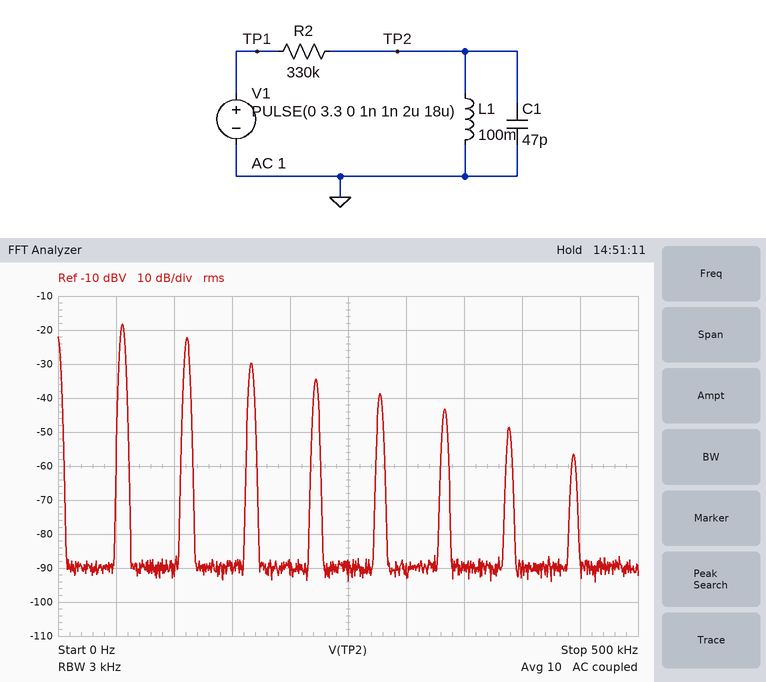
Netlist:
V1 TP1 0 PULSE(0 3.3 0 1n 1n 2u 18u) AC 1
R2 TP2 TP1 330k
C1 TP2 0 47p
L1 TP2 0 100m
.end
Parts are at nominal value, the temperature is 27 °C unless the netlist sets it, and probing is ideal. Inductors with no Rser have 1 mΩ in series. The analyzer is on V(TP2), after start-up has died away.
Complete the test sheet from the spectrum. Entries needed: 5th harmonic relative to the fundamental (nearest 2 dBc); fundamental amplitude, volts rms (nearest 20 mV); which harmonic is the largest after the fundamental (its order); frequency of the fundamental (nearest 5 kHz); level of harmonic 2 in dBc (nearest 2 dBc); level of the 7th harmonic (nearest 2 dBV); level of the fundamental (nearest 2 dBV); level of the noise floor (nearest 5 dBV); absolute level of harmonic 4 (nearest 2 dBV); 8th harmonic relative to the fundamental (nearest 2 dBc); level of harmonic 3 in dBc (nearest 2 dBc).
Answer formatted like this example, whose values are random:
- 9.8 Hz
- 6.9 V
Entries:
- -20 dBc
- 120 mV
- 2
- 55 kHz
- -4 dBc
- -48 dBV
- -18 dBV
- -90 dBV
- -34 dBV
- -38 dBc
- -12 dBc
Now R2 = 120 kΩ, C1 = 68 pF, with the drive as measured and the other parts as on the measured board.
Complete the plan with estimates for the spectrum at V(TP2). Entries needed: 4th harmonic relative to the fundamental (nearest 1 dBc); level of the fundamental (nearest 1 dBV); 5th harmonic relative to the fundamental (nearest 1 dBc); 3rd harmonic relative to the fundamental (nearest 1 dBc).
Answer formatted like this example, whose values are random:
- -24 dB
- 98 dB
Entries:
- -22 dBc
- -7 dBV
- -26 dBc
- -18 dBc
